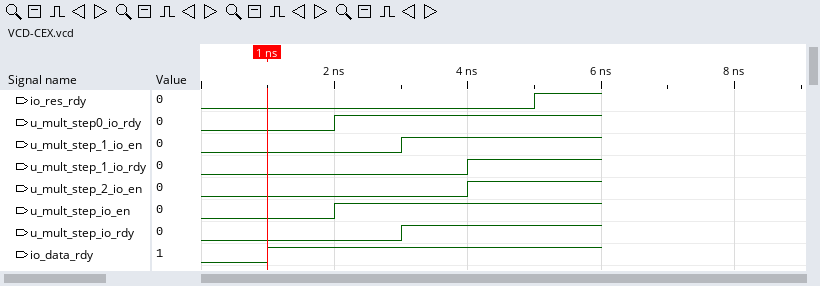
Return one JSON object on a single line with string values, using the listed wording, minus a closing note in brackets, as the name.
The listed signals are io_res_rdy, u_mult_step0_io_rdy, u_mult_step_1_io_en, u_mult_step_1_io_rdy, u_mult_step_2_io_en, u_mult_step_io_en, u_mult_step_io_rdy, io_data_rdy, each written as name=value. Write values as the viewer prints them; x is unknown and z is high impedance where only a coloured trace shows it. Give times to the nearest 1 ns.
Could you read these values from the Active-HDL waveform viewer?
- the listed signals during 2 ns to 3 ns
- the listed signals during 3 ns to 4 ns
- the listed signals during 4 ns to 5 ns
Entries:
{"the listed signals during 2 ns to 3 ns": "io_res_rdy=0, u_mult_step0_io_rdy=1, u_mult_step_1_io_en=0, u_mult_step_1_io_rdy=0, u_mult_step_2_io_en=0, u_mult_step_io_en=1, u_mult_step_io_rdy=0, io_data_rdy=1", "the listed signals during 3 ns to 4 ns": "io_res_rdy=0, u_mult_step0_io_rdy=1, u_mult_step_1_io_en=1, u_mult_step_1_io_rdy=0, u_mult_step_2_io_en=0, u_mult_step_io_en=1, u_mult_step_io_rdy=1, io_data_rdy=1", "the listed signals during 4 ns to 5 ns": "io_res_rdy=0, u_mult_step0_io_rdy=1, u_mult_step_1_io_en=1, u_mult_step_1_io_rdy=1, u_mult_step_2_io_en=1, u_mult_step_io_en=1, u_mult_step_io_rdy=1, io_data_rdy=1"}
